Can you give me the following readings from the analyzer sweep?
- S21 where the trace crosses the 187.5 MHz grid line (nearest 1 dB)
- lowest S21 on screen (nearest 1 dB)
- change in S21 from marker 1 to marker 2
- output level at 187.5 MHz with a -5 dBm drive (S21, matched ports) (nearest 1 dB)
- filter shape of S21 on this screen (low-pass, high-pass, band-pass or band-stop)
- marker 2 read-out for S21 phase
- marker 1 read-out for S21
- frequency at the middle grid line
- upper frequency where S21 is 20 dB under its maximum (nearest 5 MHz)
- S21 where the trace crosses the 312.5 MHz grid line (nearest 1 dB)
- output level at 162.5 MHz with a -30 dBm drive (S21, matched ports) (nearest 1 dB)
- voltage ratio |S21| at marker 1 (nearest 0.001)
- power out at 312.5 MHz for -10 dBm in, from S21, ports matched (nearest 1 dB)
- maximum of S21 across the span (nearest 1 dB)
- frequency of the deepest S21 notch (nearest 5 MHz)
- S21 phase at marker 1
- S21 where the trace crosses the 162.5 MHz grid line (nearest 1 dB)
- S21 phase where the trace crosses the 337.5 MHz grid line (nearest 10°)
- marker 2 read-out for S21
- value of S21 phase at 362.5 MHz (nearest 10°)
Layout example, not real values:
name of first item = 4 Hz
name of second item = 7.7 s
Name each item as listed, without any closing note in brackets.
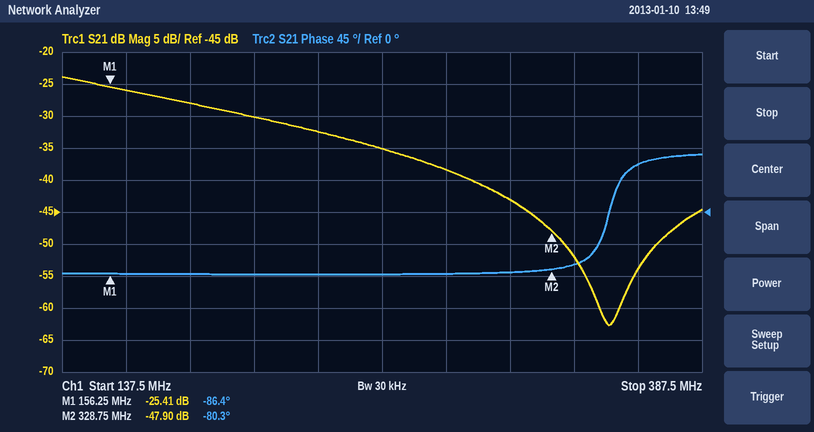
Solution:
S21 where the trace crosses the 187.5 MHz grid line = -28 dB
lowest S21 on screen = -63 dB
change in S21 from marker 1 to marker 2 = -22.49 dB
output level at 187.5 MHz with a -5 dBm drive (S21, matched ports) = -33 dBm
filter shape of S21 on this screen = low-pass
marker 2 read-out for S21 phase = -80.3°
marker 1 read-out for S21 = -25.41 dB
frequency at the middle grid line = 262.5 MHz
upper frequency where S21 is 20 dB under its maximum = 315 MHz
S21 where the trace crosses the 312.5 MHz grid line = -43 dB
output level at 162.5 MHz with a -30 dBm drive (S21, matched ports) = -56 dBm
voltage ratio |S21| at marker 1 = 0.054
power out at 312.5 MHz for -10 dBm in, from S21, ports matched = -53 dBm
maximum of S21 across the span = -24 dB
frequency of the deepest S21 notch = 350 MHz
S21 phase at marker 1 = -86.4°
S21 where the trace crosses the 162.5 MHz grid line = -26 dB
S21 phase where the trace crosses the 337.5 MHz grid line = -70°
marker 2 read-out for S21 = -47.90 dB
value of S21 phase at 362.5 MHz = 70°
